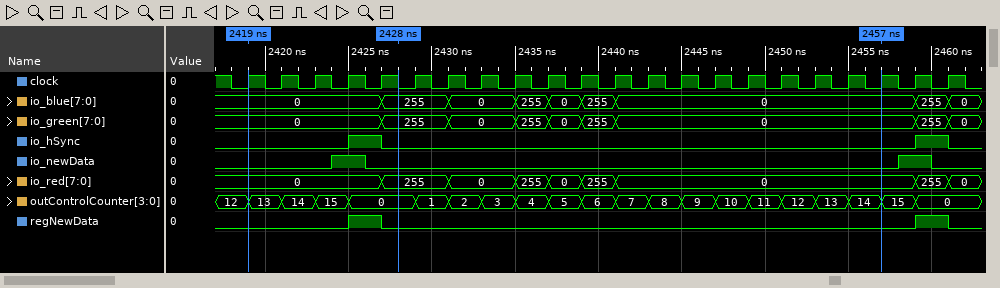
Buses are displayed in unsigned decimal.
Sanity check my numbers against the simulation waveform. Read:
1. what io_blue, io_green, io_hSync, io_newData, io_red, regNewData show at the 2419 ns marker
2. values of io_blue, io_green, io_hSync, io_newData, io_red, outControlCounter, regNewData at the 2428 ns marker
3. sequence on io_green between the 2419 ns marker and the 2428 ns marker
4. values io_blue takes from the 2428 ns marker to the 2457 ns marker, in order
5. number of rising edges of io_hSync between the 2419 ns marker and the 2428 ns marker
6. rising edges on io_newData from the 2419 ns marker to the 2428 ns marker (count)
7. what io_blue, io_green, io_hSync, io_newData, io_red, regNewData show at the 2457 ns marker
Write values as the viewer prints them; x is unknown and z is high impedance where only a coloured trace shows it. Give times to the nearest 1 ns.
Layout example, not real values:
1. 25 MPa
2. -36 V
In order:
1. io_blue=0, io_green=0, io_hSync=0, io_newData=0, io_red=0, regNewData=0
2. io_blue=255, io_green=255, io_hSync=0, io_newData=0, io_red=255, outControlCounter=0, regNewData=0
3. 0, 255
4. 255, 0, 255, 0, 255, 0
5. 1
6. 1
7. io_blue=0, io_green=0, io_hSync=0, io_newData=0, io_red=0, regNewData=0
